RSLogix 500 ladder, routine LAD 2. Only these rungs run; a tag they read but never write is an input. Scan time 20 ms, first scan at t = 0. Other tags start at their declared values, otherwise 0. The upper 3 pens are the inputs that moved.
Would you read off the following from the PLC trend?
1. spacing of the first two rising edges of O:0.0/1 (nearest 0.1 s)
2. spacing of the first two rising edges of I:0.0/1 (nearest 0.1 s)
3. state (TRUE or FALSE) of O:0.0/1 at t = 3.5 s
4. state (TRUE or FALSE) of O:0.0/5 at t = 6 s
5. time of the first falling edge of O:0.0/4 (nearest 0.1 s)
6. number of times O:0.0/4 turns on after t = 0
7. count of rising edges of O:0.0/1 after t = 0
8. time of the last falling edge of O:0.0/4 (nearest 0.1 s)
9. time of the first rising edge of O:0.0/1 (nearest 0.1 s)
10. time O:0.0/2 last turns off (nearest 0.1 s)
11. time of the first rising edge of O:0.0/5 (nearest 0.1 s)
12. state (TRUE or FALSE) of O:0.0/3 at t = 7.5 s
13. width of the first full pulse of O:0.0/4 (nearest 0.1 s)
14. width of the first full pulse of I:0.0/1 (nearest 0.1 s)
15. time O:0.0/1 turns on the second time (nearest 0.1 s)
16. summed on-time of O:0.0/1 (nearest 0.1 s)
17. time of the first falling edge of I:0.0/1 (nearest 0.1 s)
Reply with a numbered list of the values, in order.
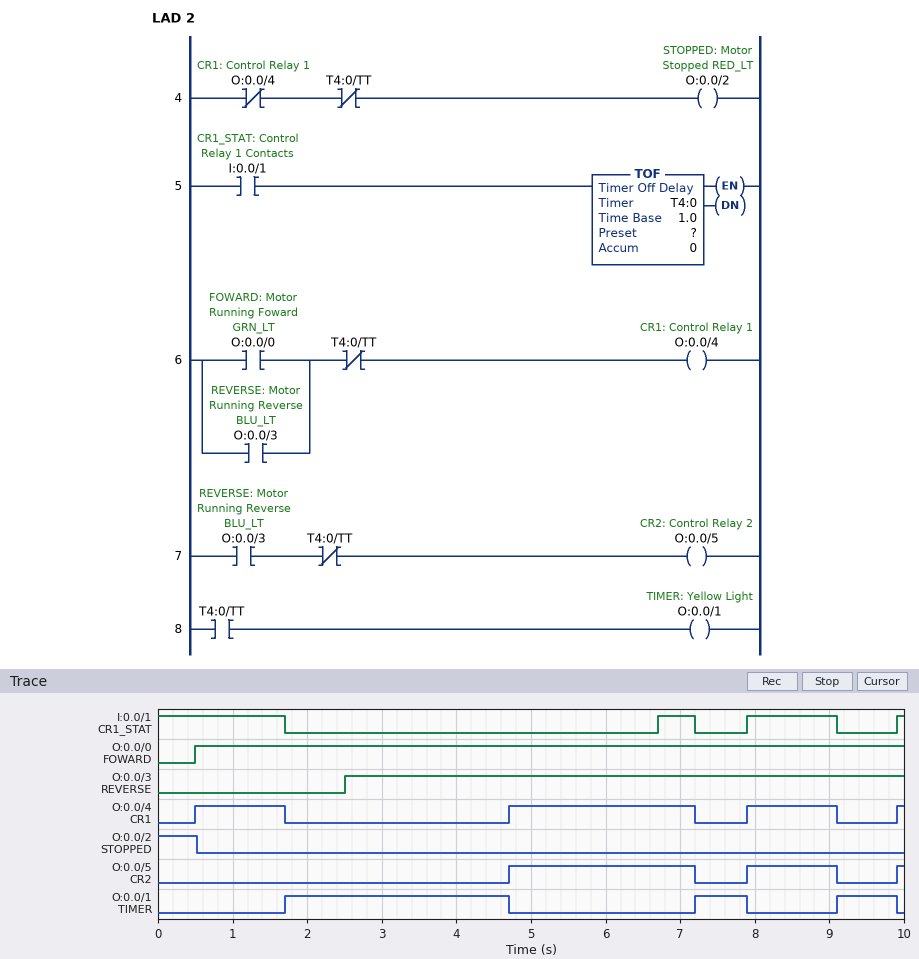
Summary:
1. 5.5 s
2. 1.2 s
3. TRUE
4. TRUE
5. 1.7 s
6. 4
7. 3
8. 9.1 s
9. 1.7 s
10. 0.5 s
11. 4.7 s
12. TRUE
13. 1.2 s
14. 0.5 s
15. 7.2 s
16. 4.5 s
17. 1.7 s
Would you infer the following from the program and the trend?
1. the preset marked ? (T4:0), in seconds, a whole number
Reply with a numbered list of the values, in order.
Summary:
1. 3 s
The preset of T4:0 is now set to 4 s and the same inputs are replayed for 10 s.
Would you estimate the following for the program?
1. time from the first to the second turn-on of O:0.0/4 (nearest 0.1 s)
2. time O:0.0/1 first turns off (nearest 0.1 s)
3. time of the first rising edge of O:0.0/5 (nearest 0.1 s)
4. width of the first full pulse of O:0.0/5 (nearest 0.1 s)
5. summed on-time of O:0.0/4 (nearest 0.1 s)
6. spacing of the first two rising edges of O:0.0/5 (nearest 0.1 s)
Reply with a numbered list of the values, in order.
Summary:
1. 5.2 s
2. 5.7 s
3. 5.7 s
4. 1.5 s
5. 4.0 s
6. 2.2 s
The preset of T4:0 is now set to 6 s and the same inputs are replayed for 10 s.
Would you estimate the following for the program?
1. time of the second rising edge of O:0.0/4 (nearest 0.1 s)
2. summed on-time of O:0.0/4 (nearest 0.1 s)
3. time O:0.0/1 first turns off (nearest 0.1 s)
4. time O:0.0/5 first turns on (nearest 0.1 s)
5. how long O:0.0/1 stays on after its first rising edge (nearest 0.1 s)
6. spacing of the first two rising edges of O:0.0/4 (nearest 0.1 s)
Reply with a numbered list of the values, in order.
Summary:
1. 6.7 s
2. 3.0 s
3. 6.7 s
4. 6.7 s
5. 5.0 s
6. 6.2 s
